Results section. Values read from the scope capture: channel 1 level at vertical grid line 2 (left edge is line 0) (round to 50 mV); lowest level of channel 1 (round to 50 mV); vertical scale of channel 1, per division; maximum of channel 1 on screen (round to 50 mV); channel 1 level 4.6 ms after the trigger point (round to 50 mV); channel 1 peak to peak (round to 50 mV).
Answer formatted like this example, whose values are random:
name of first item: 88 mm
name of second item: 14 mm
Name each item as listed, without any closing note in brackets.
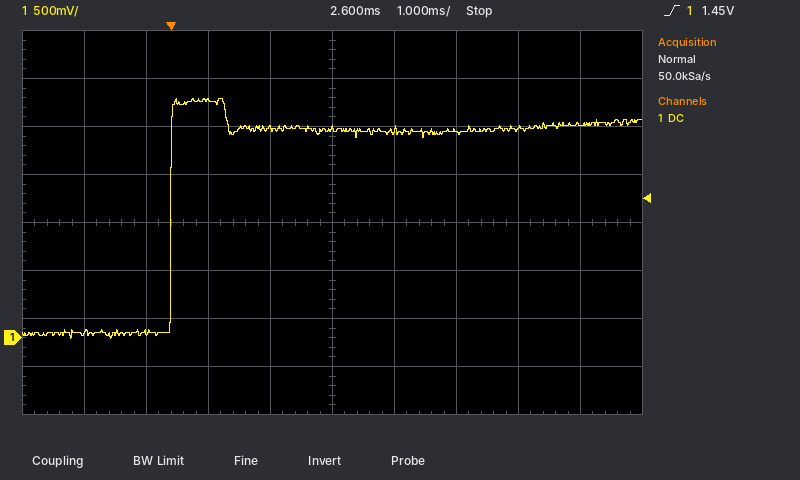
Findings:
channel 1 level at vertical grid line 2 (left edge is line 0): 50 mV
lowest level of channel 1: 0 mV
vertical scale of channel 1, per division: 500 mV
maximum of channel 1 on screen: 2.50 V
channel 1 level 4.6 ms after the trigger point: 2.15 V
channel 1 peak to peak: 2.50 V
